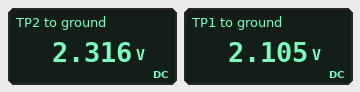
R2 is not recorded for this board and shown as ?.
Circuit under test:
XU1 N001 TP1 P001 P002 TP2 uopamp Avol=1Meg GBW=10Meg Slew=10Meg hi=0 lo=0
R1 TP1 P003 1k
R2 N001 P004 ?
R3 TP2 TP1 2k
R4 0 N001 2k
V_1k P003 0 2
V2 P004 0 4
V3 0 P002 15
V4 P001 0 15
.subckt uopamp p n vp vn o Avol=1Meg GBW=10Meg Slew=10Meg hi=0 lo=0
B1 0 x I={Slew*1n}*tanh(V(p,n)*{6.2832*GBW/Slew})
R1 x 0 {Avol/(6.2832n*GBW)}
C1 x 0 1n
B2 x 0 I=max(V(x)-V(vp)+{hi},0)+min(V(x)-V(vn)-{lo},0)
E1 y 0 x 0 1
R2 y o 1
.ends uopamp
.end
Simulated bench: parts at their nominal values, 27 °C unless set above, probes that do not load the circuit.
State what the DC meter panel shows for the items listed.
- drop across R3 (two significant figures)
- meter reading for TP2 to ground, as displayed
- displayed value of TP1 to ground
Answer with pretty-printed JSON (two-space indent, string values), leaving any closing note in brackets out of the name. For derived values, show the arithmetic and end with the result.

{
  "drop across R3": "2.316 V - 2.105 V = 210 mV",
  "meter reading for TP2 to ground, as displayed": "2.316 V",
  "displayed value of TP1 to ground": "2.105 V"
}
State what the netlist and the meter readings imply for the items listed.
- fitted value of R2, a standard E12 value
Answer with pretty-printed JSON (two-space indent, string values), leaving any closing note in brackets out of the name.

{
  "fitted value of R2, a standard E12 value": "1.8 kΩ"
}
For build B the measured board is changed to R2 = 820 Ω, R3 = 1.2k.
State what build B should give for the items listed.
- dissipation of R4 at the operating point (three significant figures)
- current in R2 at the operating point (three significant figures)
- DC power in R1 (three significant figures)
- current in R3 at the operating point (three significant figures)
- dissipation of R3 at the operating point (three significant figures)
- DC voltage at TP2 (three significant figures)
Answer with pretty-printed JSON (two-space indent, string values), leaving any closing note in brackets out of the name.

{
  "dissipation of R4 at the operating point": "4.02 mW",
  "current in R2 at the operating point": "1.42 mA",
  "DC power in R1": "700 µW",
  "current in R3 at the operating point": "837 µA",
  "dissipation of R3 at the operating point": "840 µW",
  "DC voltage at TP2": "3.84 V"
}
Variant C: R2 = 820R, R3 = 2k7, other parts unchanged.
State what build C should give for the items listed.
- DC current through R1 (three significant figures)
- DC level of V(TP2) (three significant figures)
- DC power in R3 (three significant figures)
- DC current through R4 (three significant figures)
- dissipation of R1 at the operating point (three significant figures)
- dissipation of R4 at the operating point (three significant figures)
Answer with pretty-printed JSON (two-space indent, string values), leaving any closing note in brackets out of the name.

{
  "DC current through R1": "837 µA",
  "DC level of V(TP2)": "5.10 V",
  "DC power in R3": "1.89 mW",
  "DC current through R4": "1.42 mA",
  "dissipation of R1 at the operating point": "700 µW",
  "dissipation of R4 at the operating point": "4.02 mW"
}
